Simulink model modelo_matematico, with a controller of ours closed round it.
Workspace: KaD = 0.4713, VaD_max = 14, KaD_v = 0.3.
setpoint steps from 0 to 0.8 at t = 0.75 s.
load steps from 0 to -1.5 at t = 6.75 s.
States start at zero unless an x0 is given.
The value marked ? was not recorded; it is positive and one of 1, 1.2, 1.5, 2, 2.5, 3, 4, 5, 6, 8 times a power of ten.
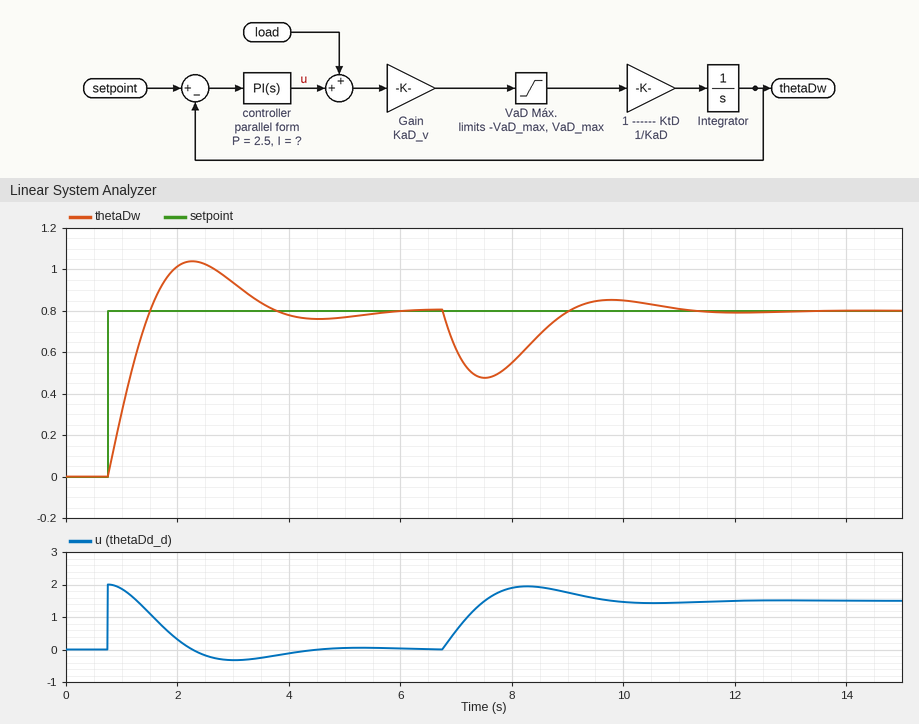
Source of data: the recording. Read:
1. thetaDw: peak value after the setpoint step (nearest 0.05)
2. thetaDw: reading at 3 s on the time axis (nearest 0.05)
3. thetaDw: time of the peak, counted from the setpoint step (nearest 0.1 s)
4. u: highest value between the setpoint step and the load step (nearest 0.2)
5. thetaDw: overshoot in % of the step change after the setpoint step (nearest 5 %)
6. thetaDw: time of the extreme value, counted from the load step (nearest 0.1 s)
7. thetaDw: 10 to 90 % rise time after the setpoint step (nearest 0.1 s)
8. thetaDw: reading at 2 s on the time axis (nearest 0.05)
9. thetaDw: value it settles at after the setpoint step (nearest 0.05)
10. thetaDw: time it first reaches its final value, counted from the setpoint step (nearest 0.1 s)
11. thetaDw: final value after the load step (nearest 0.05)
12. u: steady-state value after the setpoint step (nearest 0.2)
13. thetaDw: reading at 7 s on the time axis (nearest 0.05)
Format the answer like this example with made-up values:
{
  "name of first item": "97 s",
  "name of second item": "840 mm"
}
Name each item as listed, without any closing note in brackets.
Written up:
{
  "thetaDw: peak value after the setpoint step": "1.05",
  "thetaDw: reading at 3 s on the time axis": "0.95",
  "thetaDw: time of the peak, counted from the setpoint step": "1.5 s",
  "u: highest value between the setpoint step and the load step": "2.0",
  "thetaDw: overshoot in % of the step change after the setpoint step": "30 %",
  "thetaDw: time of the extreme value, counted from the load step": "0.8 s",
  "thetaDw: 10 to 90 % rise time after the setpoint step": "0.6 s",
  "thetaDw: reading at 2 s on the time axis": "1.00",
  "thetaDw: value it settles at after the setpoint step": "0.80",
  "thetaDw: time it first reaches its final value, counted from the setpoint step": "0.8 s",
  "thetaDw: final value after the load step": "0.80",
  "u: steady-state value after the setpoint step": "0.0",
  "thetaDw: reading at 7 s on the time axis": "0.60"
}
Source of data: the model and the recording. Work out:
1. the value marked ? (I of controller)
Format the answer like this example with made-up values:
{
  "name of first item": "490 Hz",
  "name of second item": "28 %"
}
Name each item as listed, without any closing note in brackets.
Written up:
{
  "the value marked ?": "4"
}
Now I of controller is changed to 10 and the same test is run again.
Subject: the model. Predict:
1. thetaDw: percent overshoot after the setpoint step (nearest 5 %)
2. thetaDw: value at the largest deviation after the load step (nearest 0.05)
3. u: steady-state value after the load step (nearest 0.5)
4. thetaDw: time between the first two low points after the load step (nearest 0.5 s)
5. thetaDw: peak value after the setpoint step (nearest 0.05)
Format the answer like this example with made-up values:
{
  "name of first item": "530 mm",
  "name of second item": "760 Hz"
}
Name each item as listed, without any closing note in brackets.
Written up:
{
  "thetaDw: percent overshoot after the setpoint step": "45 %",
  "thetaDw: value at the largest deviation after the load step": "0.55",
  "u: steady-state value after the load step": "1.5",
  "thetaDw: time between the first two low points after the load step": "2.5 s",
  "thetaDw: peak value after the setpoint step": "1.15"
}
